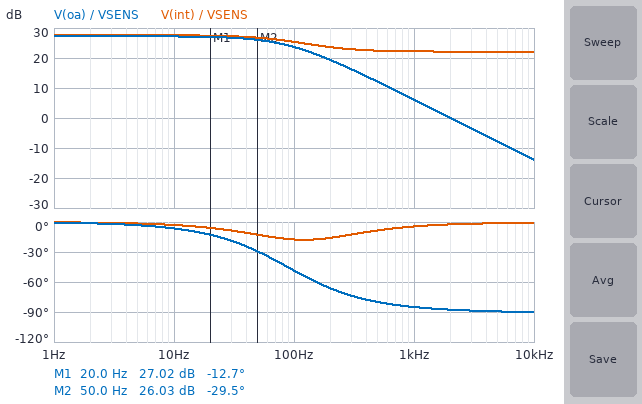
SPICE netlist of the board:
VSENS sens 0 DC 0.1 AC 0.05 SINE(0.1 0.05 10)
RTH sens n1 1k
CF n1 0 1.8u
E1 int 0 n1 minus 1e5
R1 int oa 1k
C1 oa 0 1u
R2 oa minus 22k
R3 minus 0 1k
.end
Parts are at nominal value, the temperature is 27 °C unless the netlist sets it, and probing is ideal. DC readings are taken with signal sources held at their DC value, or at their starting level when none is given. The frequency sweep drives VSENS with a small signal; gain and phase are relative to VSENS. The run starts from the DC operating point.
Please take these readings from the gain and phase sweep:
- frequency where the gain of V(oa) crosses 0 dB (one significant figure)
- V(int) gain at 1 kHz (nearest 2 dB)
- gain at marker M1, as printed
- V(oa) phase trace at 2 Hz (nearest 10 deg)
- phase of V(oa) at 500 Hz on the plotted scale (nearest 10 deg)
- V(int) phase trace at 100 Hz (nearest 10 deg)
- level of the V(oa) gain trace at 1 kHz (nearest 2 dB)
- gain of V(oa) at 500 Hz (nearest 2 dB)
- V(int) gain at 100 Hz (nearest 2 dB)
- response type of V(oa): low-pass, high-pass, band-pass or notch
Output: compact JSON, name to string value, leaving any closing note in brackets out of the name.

{"frequency where the gain of V(oa) crosses 0 dB": "2 kHz", "V(int) gain at 1 kHz": "22 dB", "gain at marker M1, as printed": "27.02 dB", "V(oa) phase trace at 2 Hz": "0 deg", "phase of V(oa) at 500 Hz on the plotted scale": "-80 deg", "V(int) phase trace at 100 Hz": "-20 deg", "level of the V(oa) gain trace at 1 kHz": "6 dB", "gain of V(oa) at 500 Hz": "12 dB", "V(int) gain at 100 Hz": "26 dB", "response type of V(oa): low-pass, high-pass, band-pass or notch": "low-pass"}
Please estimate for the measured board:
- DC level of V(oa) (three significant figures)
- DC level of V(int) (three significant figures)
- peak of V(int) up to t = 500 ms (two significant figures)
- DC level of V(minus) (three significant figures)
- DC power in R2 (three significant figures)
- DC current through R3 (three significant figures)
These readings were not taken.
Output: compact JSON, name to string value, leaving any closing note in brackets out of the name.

{"DC level of V(oa)": "2.30 V", "DC level of V(int)": "2.40 V", "peak of V(int) up to t = 500 ms": "3.6 V", "DC level of V(minus)": "100 mV", "DC power in R2": "220 µW", "DC current through R3": "100 µA"}
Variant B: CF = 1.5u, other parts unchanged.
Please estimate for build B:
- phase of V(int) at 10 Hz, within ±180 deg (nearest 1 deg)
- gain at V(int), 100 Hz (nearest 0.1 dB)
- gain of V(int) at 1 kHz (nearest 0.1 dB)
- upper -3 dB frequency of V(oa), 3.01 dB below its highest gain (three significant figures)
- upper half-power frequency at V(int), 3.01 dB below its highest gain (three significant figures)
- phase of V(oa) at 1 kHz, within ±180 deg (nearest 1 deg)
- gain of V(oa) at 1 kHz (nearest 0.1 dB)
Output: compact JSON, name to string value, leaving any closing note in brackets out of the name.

{"phase of V(int) at 10 Hz, within ±180 deg": "-2 deg", "gain at V(int), 100 Hz": "26.2 dB", "gain of V(int) at 1 kHz": "23.8 dB", "upper -3 dB frequency of V(oa), 3.01 dB below its highest gain": "106 Hz", "upper half-power frequency at V(int), 3.01 dB below its highest gain": "248 Hz", "phase of V(oa) at 1 kHz, within ±180 deg": "-84 deg", "gain of V(oa) at 1 kHz": "7.7 dB"}
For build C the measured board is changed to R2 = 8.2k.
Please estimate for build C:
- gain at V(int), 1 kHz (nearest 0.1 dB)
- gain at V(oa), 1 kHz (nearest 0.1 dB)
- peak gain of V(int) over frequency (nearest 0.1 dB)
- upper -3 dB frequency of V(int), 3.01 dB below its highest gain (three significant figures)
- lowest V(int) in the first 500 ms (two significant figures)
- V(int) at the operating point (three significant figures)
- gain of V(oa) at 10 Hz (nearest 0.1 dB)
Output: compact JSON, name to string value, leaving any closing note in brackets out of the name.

{"gain at V(int), 1 kHz": "14.3 dB", "gain at V(oa), 1 kHz": "-1.8 dB", "peak gain of V(int) over frequency": "20.2 dB", "upper -3 dB frequency of V(int), 3.01 dB below its highest gain": "125 Hz", "lowest V(int) in the first 500 ms": "510 mV", "V(int) at the operating point": "1.02 V", "gain of V(oa) at 10 Hz": "19.2 dB"}
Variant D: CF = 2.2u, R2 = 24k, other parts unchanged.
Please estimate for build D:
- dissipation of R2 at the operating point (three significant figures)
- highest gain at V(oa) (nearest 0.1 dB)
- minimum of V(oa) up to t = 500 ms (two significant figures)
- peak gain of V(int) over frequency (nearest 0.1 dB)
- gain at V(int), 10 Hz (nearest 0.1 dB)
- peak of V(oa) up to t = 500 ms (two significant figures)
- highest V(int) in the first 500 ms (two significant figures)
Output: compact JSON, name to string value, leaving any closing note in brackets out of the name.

{"dissipation of R2 at the operating point": "240 µW", "highest gain at V(oa)": "28.0 dB", "minimum of V(oa) up to t = 500 ms": "1.3 V", "peak gain of V(int) over frequency": "28.3 dB", "gain at V(int), 10 Hz": "28.2 dB", "peak of V(oa) up to t = 500 ms": "3.7 V", "highest V(int) in the first 500 ms": "3.9 V"}
